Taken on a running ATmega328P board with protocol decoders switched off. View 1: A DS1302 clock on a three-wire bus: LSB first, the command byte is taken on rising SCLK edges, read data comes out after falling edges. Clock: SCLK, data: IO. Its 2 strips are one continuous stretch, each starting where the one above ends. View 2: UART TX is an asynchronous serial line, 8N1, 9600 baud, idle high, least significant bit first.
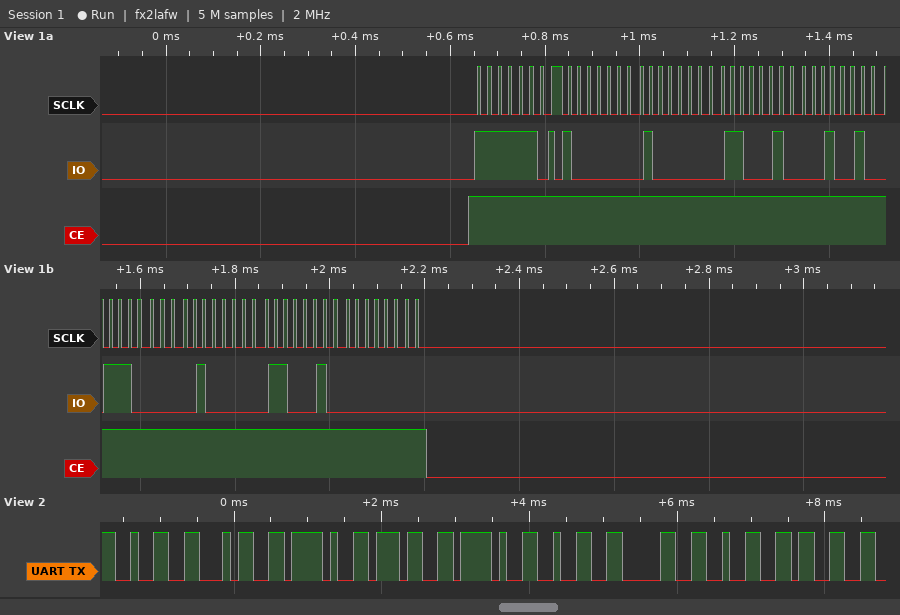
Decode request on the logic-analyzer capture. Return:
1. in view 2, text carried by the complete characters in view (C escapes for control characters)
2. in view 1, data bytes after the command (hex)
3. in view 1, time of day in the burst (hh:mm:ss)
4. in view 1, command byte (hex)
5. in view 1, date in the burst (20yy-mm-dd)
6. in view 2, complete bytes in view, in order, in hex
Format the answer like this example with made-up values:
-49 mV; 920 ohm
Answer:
"24/7/2023"; 01 01 23 24 07 02 23 00; 23:01:01; 0xBF; 2023-07-24; 32 34 2F 37 2F 32 30 32 33
